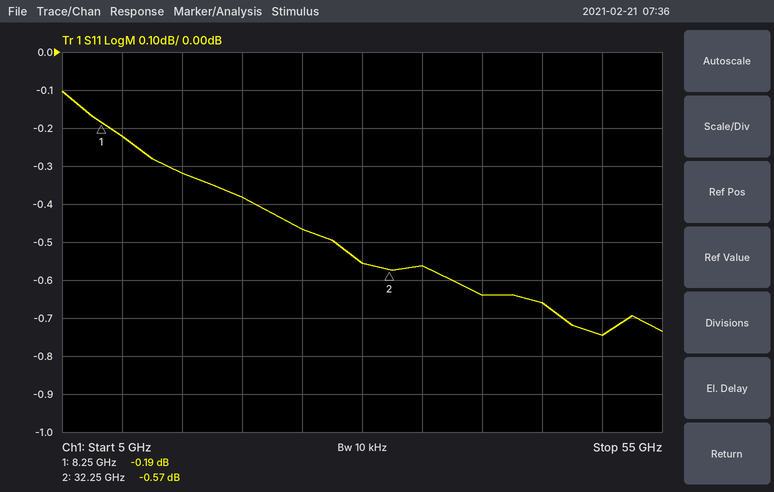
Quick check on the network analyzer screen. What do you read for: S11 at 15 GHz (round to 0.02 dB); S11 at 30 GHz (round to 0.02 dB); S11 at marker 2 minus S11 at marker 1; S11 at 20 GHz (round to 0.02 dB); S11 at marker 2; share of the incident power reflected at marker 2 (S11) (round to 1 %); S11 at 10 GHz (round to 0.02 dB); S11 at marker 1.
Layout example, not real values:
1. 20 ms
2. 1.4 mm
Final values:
1. -0.32 dB
2. -0.56 dB
3. -0.38 dB
4. -0.38 dB
5. -0.57 dB
6. 88 %
7. -0.22 dB
8. -0.19 dB
